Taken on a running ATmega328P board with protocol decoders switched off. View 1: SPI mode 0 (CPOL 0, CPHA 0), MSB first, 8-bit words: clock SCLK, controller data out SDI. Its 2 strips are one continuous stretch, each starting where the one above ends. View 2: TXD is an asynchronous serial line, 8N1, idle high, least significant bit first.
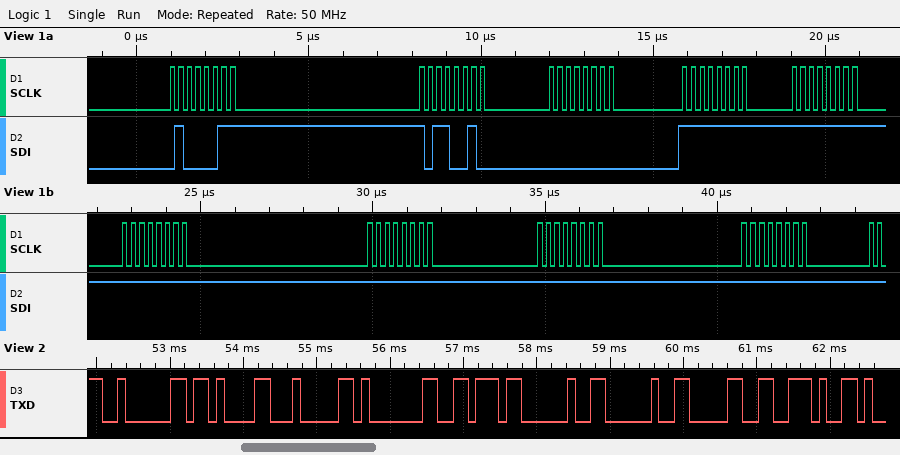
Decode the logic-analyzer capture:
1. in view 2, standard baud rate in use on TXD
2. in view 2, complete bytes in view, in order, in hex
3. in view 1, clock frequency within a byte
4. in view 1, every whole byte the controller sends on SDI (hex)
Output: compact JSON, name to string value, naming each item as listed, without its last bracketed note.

{"in view 2, standard baud rate in use on TXD": "9600 baud", "in view 2, complete bytes in view, in order, in hex": "0x02 0x0B 0x04 0x01 0x76 0x20 0x20 0x30 0x2E", "in view 1, clock frequency within a byte": "4 MHz", "in view 1, every whole byte the controller sends on SDI": "43 B2 00 FF FF FF FF FF FF"}
